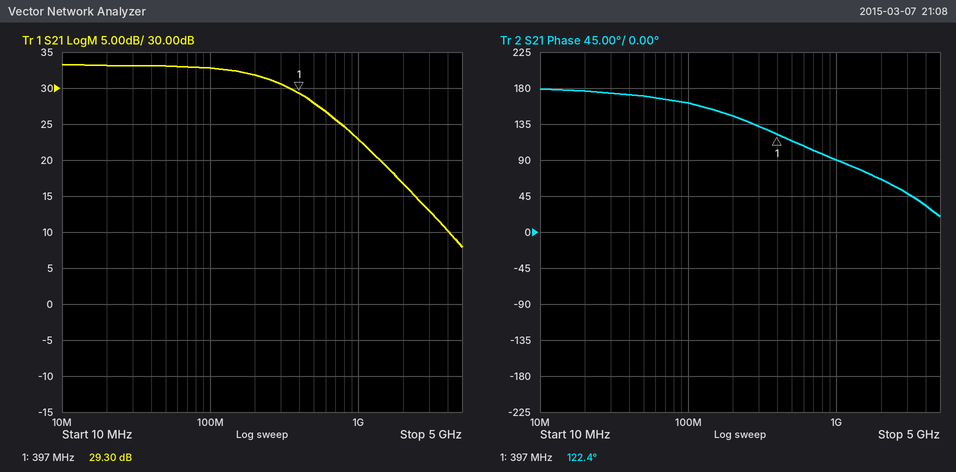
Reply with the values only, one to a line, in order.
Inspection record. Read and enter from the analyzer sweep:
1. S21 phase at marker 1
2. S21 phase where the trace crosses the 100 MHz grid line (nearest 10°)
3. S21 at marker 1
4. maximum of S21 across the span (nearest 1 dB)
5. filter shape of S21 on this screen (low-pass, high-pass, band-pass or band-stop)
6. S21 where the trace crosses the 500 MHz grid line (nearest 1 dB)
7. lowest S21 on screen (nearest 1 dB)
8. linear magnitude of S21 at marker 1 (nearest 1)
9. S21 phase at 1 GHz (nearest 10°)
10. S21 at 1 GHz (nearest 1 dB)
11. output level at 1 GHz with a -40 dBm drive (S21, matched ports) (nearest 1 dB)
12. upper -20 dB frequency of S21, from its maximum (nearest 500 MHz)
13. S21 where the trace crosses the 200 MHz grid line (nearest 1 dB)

122.4°
160°
29.30 dB
33 dB
low-pass
28 dB
8 dB
29
90°
23 dB
-17 dBm
3.0 GHz
32 dB
